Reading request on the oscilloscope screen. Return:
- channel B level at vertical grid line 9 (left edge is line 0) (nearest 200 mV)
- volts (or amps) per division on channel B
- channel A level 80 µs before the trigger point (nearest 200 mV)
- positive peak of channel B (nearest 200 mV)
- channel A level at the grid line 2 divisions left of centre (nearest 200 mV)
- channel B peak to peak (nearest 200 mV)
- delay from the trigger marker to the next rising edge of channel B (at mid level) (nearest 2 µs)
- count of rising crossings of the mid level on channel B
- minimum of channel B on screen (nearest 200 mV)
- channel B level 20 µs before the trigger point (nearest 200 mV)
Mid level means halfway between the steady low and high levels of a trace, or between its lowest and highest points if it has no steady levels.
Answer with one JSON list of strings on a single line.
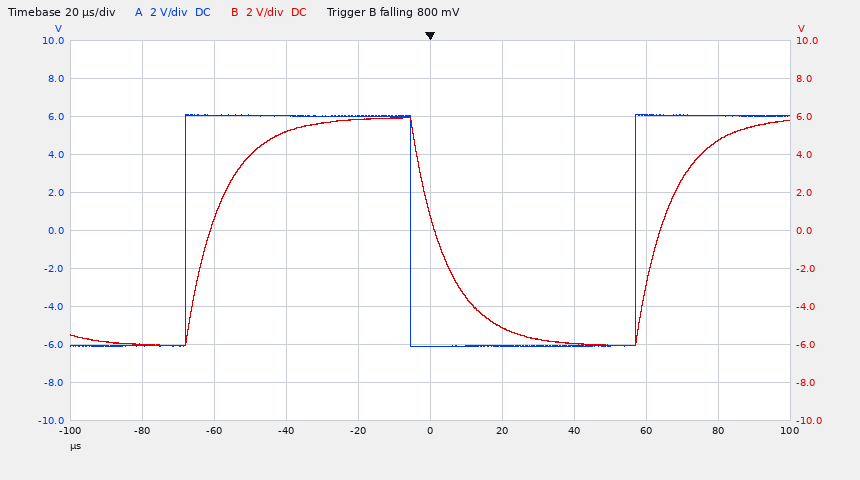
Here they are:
["4.8 V", "2 V", "-6.0 V", "6.0 V", "6.0 V", "12.0 V", "64 µs", "2", "-6.0 V", "5.8 V"]
